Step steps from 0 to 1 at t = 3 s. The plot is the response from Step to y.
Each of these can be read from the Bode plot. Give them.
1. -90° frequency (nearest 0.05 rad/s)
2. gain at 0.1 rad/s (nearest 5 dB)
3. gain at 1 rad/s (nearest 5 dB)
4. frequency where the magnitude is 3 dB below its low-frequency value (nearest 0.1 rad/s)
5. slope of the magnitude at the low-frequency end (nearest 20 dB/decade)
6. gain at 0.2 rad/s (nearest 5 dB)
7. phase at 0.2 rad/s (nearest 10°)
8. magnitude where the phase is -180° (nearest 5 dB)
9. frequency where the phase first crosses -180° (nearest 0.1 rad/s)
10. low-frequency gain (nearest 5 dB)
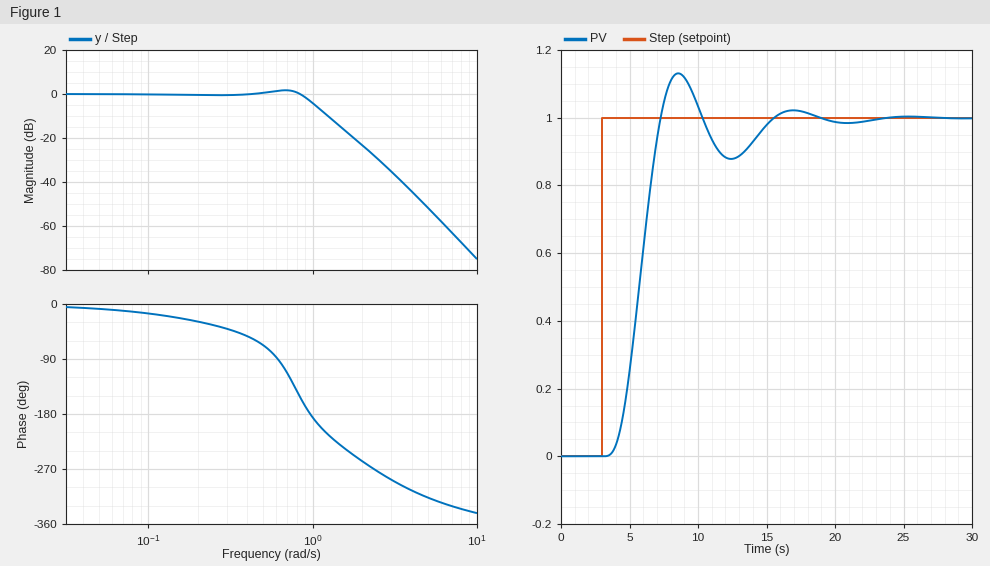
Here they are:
0.60 rad/s
0 dB
-5 dB
1.0 rad/s
0 dB/decade
0 dB
-30°
-5 dB
1.0 rad/s
0 dB
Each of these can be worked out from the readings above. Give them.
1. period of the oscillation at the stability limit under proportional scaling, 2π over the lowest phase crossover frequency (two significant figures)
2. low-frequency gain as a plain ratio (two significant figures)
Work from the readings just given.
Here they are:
6.3 s
1.0
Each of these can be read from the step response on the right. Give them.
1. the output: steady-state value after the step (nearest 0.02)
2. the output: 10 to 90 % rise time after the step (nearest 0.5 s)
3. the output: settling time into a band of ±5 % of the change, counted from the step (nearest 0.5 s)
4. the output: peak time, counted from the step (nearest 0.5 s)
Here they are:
1.00
2.5 s
11.5 s
5.5 s
